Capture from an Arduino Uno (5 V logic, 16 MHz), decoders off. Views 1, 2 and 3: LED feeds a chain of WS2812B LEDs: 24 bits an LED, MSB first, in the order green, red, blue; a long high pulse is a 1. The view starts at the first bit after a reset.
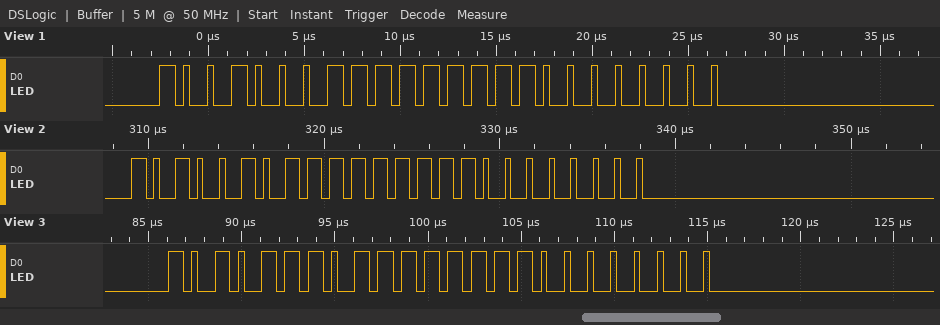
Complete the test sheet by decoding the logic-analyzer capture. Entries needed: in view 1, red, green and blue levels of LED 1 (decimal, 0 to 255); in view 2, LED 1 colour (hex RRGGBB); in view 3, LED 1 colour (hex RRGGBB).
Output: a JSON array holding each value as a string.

["255, 145, 0", "#FFA500", "#FFAE00"]
